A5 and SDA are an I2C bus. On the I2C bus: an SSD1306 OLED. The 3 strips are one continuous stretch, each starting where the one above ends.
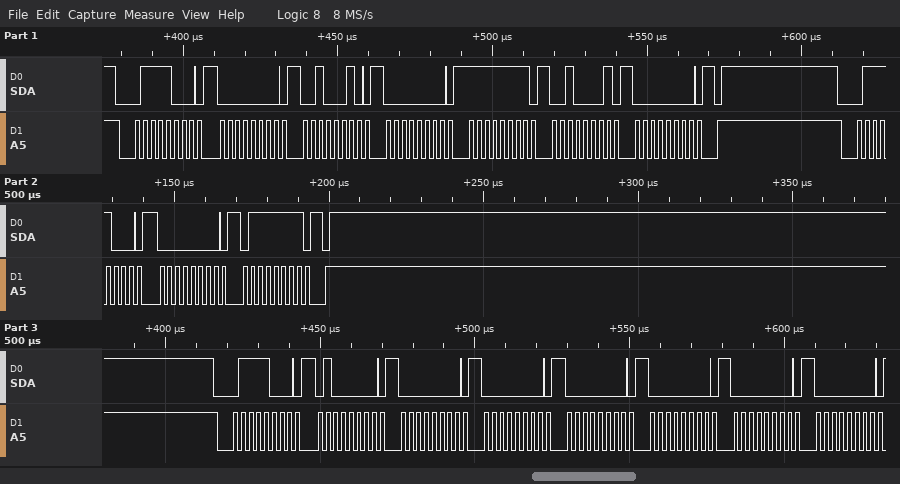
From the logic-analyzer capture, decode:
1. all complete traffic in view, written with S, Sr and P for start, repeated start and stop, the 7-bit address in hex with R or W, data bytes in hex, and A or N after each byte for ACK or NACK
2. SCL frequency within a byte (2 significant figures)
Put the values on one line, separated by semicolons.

S 3CW A 00 A 22 A 00 A FF A 21 A 00 A P S 3CW A 00 A 7F A P S 3CW A 40 A 00 A 00 A 00 A 00 A 00 A 00 A; 400 kHz
